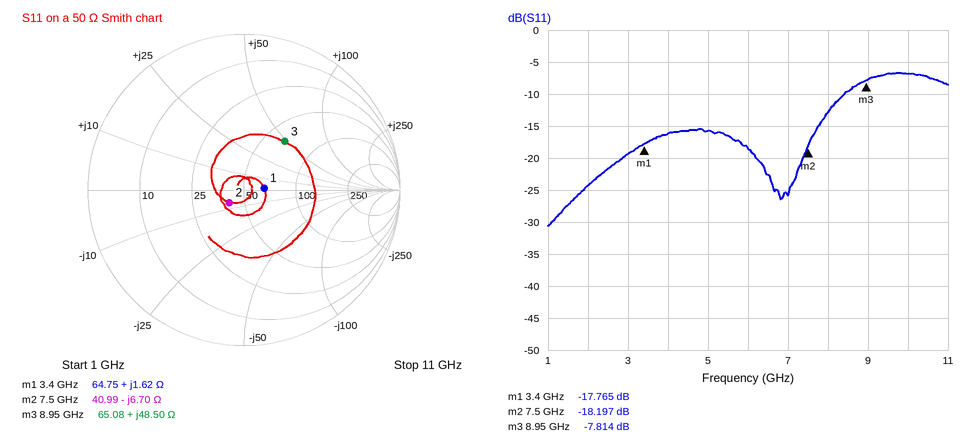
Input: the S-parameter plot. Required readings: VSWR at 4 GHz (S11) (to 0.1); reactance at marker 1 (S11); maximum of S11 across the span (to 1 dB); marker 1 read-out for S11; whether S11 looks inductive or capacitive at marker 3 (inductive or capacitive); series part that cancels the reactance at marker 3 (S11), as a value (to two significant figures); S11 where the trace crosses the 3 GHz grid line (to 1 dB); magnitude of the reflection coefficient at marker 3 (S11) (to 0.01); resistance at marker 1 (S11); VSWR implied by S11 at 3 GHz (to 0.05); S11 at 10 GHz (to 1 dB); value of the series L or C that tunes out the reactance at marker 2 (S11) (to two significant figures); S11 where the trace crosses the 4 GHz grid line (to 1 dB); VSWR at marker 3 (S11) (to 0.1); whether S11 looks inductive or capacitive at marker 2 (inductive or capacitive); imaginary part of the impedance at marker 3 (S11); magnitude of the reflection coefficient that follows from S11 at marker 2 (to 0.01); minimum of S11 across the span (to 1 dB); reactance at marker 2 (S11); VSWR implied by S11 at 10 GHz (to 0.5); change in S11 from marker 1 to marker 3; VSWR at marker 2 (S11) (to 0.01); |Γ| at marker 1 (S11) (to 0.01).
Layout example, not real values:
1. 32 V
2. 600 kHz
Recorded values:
1. 1.4
2. +1.62 Ω
3. -7 dB
4. -17.765 dB
5. inductive
6. 370 fF
7. -19 dB
8. 0.41
9. 64.75 Ω
10. 1.25
11. -7 dB
12. 140 pH
13. -16 dB
14. 2.4
15. capacitive
16. +48.50 Ω
17. 0.12
18. -31 dB
19. -6.70 Ω
20. 2.5
21. 9.951 dB
22. 1.28
23. 0.13
